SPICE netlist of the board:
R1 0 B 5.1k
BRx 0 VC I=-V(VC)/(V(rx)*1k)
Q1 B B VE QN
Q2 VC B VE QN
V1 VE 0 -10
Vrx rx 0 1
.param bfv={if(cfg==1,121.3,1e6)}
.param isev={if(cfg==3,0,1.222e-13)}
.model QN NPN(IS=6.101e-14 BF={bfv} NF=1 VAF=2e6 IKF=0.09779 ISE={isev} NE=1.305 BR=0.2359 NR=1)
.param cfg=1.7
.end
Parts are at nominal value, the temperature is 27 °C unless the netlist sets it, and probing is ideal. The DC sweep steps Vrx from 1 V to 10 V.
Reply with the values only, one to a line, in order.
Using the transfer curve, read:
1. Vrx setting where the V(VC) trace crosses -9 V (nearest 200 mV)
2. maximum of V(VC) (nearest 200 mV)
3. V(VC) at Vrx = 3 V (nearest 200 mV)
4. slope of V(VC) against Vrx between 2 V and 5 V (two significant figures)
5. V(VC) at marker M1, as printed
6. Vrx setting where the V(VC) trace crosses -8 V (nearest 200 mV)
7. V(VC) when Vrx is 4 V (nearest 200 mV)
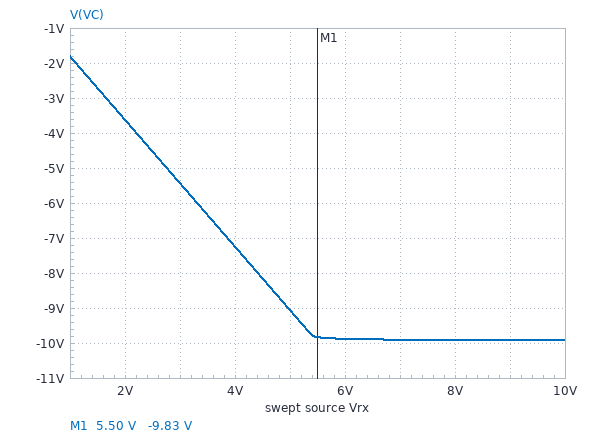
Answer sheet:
5.0 V
-1.8 V
-5.4 V
-1.8 V/V
-9.83 V
4.4 V
-7.2 V
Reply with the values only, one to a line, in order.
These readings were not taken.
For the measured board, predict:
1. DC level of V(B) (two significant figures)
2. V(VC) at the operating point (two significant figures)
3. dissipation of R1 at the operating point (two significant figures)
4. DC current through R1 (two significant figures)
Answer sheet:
-9.4 V
-1.8 V
17 mW
1.8 mA
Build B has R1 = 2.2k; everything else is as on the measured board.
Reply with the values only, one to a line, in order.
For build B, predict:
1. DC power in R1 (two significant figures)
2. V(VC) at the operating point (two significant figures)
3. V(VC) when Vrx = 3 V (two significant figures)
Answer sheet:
40 mW
-4.2 V
-9.9 V
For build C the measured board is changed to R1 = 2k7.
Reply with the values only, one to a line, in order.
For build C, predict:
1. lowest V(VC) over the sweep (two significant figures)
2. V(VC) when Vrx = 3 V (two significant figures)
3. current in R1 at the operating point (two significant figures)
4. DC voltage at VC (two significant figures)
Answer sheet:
-9.9 V
-9.9 V
3.5 mA
-3.4 V
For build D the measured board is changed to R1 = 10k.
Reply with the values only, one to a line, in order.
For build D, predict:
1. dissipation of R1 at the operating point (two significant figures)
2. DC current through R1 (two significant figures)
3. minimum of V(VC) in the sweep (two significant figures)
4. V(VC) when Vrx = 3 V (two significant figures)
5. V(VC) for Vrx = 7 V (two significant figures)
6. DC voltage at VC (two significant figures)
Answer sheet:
8.8 mW
940 µA
-9.2 V
-2.8 V
-6.5 V
-920 mV
